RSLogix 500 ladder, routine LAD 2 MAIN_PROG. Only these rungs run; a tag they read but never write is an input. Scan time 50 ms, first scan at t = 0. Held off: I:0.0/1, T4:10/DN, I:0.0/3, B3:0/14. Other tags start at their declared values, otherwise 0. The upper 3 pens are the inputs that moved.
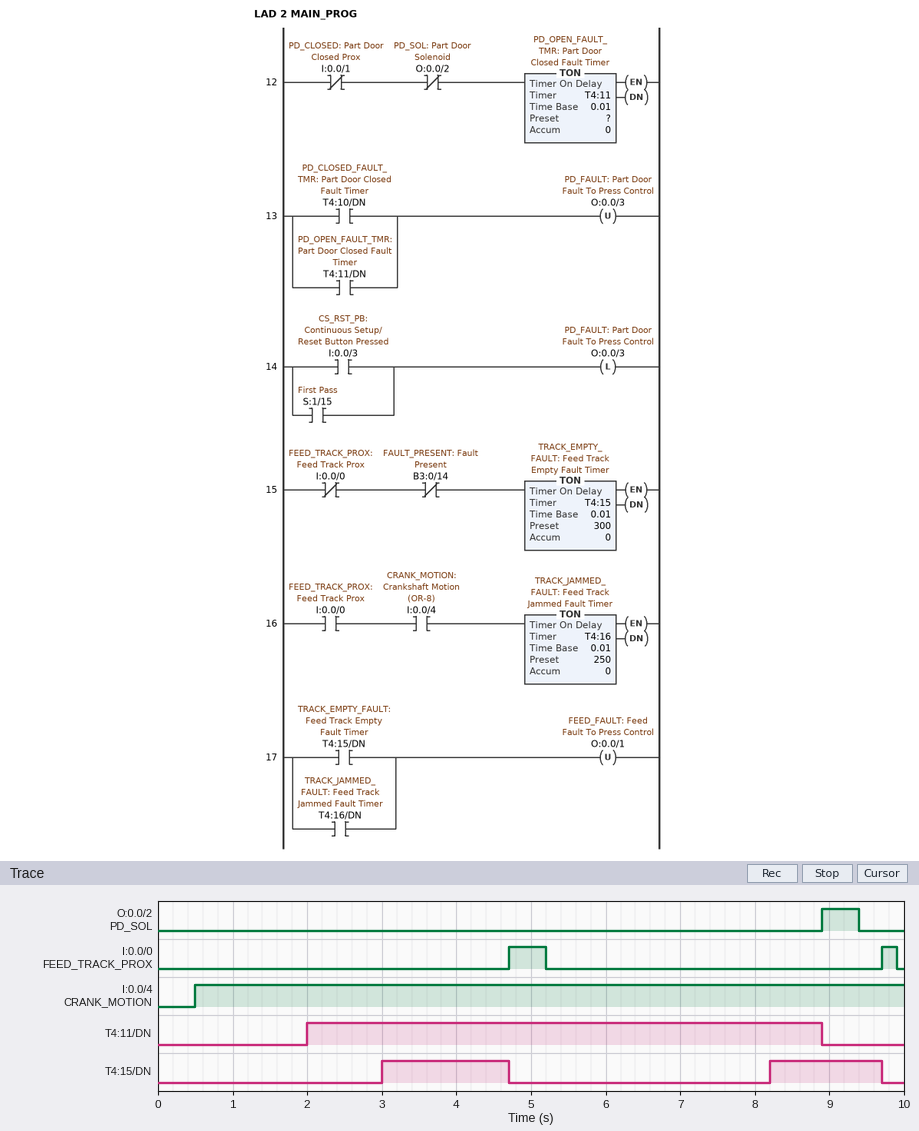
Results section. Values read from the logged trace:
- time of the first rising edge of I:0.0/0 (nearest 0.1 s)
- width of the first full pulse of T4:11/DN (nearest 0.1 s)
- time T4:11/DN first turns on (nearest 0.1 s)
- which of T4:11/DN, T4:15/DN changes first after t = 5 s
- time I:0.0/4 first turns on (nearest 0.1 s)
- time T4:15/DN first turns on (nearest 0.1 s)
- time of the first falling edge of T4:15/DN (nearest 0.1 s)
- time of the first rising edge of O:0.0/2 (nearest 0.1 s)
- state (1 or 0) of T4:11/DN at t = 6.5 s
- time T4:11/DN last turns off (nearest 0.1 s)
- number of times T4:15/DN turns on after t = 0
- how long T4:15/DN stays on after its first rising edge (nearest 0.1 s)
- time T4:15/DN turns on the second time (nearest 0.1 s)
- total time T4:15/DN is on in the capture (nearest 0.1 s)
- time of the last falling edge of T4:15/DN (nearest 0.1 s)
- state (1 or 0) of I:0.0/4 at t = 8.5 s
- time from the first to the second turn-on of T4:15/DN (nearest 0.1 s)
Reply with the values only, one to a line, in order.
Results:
4.7 s
6.9 s
2.0 s
T4:15/DN
0.5 s
3.0 s
4.7 s
8.9 s
1
8.9 s
2
1.7 s
8.2 s
3.2 s
9.7 s
1
5.2 s
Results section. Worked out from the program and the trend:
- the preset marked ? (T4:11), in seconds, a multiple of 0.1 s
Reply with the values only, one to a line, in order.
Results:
2.0 s
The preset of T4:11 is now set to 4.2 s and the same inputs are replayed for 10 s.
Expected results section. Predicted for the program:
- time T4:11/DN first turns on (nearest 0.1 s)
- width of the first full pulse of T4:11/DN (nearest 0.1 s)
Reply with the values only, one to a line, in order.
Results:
4.2 s
4.7 s
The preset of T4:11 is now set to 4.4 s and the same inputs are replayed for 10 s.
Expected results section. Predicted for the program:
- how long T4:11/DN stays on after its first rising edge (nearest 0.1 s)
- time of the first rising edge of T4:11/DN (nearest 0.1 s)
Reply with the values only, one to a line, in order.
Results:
4.5 s
4.4 s
